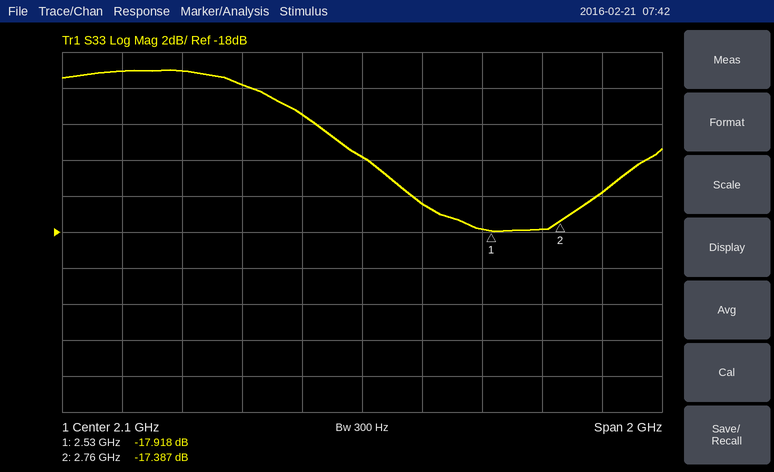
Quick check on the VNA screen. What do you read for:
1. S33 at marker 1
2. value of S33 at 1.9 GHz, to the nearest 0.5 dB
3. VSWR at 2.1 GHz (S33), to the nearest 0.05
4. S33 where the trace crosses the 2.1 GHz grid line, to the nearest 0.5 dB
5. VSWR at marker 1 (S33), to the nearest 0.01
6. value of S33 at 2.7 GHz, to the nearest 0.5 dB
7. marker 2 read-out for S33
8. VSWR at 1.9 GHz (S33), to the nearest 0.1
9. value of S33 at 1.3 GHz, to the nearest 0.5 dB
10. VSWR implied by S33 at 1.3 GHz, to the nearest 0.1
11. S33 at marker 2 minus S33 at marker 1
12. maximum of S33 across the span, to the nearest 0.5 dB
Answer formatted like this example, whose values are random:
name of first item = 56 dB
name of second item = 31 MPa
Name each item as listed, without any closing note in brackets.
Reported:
S33 at marker 1 = -17.918 dB
value of S33 at 1.9 GHz, to the nearest 0.5 dB = -11.5 dB
VSWR at 2.1 GHz (S33), to the nearest 0.05 = 1.50
S33 where the trace crosses the 2.1 GHz grid line, to the nearest 0.5 dB = -14.0 dB
VSWR at marker 1 (S33), to the nearest 0.01 = 1.29
value of S33 at 2.7 GHz, to the nearest 0.5 dB = -18.0 dB
marker 2 read-out for S33 = -17.387 dB
VSWR at 1.9 GHz (S33), to the nearest 0.1 = 1.7
value of S33 at 1.3 GHz, to the nearest 0.5 dB = -9.0 dB
VSWR implied by S33 at 1.3 GHz, to the nearest 0.1 = 2.1
S33 at marker 2 minus S33 at marker 1 = 0.531 dB
maximum of S33 across the span, to the nearest 0.5 dB = -9.0 dB
